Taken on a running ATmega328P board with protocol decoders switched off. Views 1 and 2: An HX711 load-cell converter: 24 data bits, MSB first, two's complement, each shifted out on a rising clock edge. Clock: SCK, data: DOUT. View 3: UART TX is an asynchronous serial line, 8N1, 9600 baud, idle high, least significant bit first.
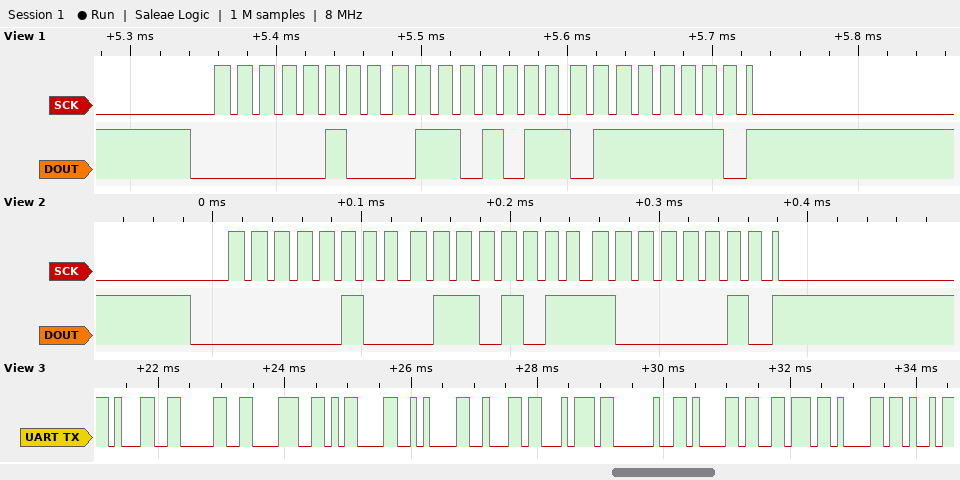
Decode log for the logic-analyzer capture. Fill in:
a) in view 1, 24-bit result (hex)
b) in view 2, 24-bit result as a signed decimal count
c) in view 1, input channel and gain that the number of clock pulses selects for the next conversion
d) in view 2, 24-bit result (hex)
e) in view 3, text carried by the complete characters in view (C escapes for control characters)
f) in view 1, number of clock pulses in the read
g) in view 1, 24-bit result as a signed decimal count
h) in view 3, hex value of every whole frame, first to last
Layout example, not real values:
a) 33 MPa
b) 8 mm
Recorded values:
a) 0x046B7E
b) 289666
c) channel A, gain 128
d) 0x046B82
e) "108\r\nbt ava"
f) 25
g) 289662
h) 31 30 38 0D 0A 62 74 20 61 76 61
